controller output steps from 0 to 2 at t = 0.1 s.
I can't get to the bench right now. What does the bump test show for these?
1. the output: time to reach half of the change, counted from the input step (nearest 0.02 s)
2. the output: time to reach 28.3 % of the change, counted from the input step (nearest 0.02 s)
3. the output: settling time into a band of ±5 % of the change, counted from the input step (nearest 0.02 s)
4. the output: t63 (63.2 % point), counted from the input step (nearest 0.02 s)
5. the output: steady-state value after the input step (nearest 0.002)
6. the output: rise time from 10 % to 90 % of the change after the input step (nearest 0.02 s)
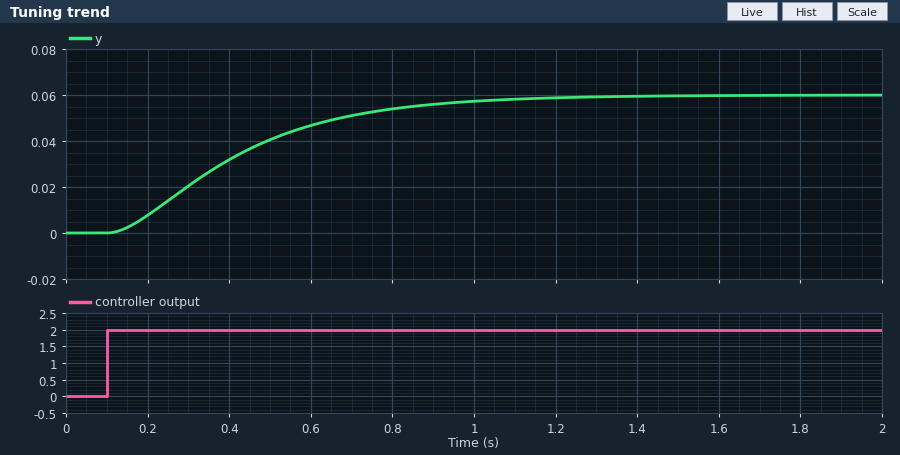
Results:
0.28 s
0.18 s
0.88 s
0.36 s
0.060
0.62 s
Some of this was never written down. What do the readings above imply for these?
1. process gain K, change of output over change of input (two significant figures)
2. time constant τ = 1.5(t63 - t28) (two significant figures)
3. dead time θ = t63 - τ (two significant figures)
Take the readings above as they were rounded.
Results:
0.030
0.27 s
0.090 s
